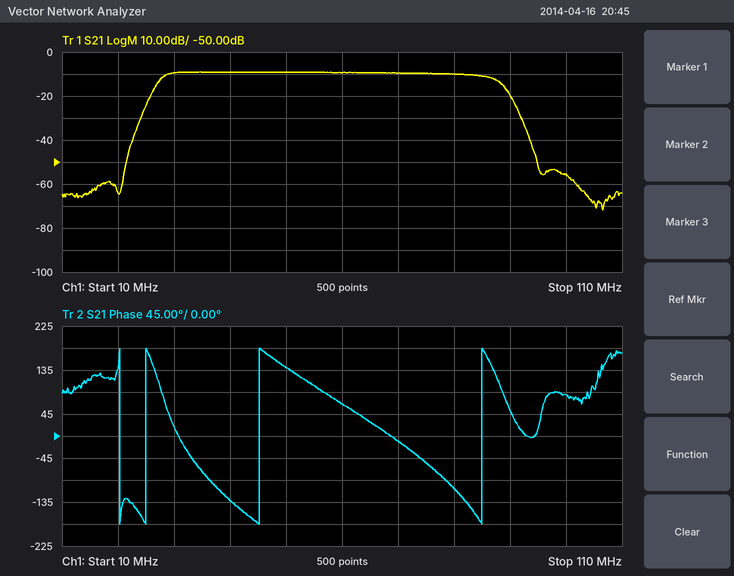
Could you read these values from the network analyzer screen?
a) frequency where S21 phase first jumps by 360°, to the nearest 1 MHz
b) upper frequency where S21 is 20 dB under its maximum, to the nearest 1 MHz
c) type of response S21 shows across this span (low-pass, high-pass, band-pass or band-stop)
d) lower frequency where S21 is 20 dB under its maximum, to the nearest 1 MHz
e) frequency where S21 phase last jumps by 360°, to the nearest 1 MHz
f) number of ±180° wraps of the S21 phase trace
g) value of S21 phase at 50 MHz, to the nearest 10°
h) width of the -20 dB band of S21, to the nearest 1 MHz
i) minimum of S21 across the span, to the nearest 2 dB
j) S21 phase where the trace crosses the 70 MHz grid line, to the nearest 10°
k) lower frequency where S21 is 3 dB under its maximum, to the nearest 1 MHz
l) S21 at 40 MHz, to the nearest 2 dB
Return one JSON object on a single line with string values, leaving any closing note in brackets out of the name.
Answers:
{"frequency where S21 phase first jumps by 360°, to the nearest 1 MHz": "20 MHz", "upper frequency where S21 is 20 dB under its maximum, to the nearest 1 MHz": "92 MHz", "type of response S21 shows across this span": "band-pass", "lower frequency where S21 is 20 dB under its maximum, to the nearest 1 MHz": "24 MHz", "frequency where S21 phase last jumps by 360°, to the nearest 1 MHz": "85 MHz", "number of ±180° wraps of the S21 phase trace": "4", "value of S21 phase at 50 MHz, to the nearest 10°": "140°", "width of the -20 dB band of S21, to the nearest 1 MHz": "68 MHz", "minimum of S21 across the span, to the nearest 2 dB": "-72 dB", "S21 phase where the trace crosses the 70 MHz grid line, to the nearest 10°": "-10°", "lower frequency where S21 is 3 dB under its maximum, to the nearest 1 MHz": "28 MHz", "S21 at 40 MHz, to the nearest 2 dB": "-10 dB"}
